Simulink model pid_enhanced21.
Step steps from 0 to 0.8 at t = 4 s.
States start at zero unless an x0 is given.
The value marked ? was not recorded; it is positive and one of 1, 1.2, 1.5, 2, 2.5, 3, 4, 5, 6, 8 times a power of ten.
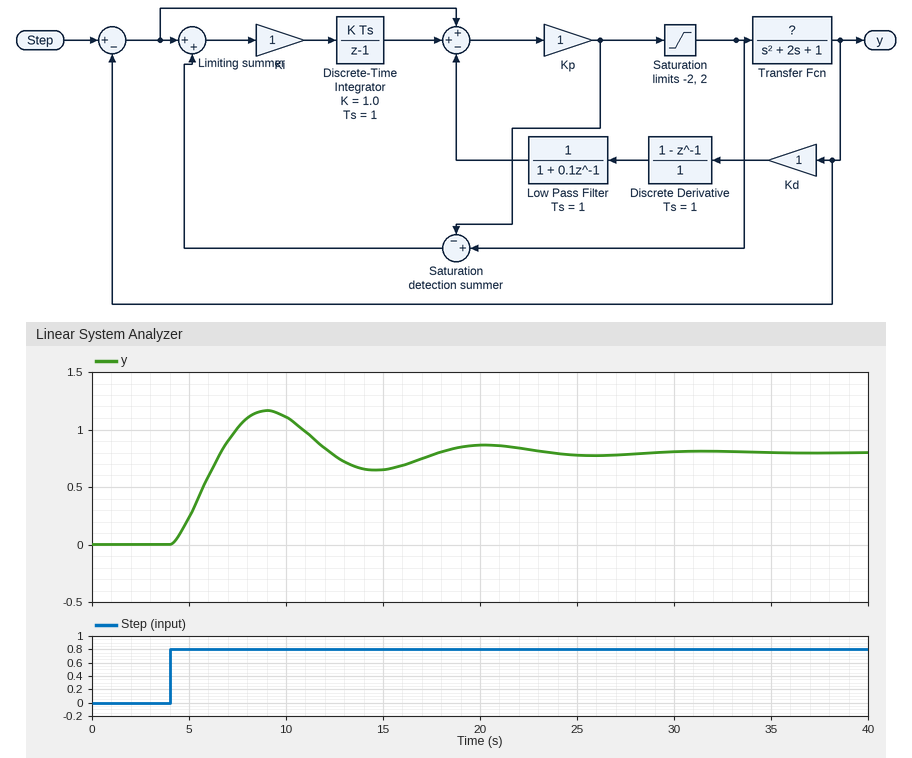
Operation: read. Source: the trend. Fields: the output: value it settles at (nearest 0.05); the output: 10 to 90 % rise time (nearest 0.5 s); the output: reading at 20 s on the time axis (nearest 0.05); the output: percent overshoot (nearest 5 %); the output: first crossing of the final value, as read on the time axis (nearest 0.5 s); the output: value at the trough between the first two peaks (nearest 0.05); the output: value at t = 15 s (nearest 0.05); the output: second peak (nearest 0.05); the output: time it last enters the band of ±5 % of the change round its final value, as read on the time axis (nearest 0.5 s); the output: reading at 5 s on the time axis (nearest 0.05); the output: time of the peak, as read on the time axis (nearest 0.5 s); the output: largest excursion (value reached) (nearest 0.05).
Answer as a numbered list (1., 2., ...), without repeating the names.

1. 0.80
2. 2.0 s
3. 0.85
4. 45 %
5. 6.5 s
6. 0.65
7. 0.65
8. 0.85
9. 22.0 s
10. 0.25
11. 9.0 s
12. 1.15
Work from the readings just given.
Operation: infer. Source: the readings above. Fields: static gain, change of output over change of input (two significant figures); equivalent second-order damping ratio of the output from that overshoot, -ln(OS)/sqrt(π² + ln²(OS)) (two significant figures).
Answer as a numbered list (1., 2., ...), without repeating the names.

1. 1.0
2. 0.25
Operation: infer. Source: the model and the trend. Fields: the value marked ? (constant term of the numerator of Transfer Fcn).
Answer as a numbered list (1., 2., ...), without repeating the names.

1. 1.2
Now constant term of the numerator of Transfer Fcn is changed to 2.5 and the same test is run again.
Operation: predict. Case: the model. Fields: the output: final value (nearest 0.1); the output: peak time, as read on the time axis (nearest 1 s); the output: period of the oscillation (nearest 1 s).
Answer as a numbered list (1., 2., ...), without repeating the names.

1. 0.8
2. 8 s
3. 9 s
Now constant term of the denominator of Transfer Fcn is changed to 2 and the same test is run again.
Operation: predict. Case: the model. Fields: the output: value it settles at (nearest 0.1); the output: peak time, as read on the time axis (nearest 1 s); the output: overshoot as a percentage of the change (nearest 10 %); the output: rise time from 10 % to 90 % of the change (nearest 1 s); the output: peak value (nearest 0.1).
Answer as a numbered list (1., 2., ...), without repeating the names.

1. 0.8
2. 10 s
3. 20 %
4. 3 s
5. 0.9
